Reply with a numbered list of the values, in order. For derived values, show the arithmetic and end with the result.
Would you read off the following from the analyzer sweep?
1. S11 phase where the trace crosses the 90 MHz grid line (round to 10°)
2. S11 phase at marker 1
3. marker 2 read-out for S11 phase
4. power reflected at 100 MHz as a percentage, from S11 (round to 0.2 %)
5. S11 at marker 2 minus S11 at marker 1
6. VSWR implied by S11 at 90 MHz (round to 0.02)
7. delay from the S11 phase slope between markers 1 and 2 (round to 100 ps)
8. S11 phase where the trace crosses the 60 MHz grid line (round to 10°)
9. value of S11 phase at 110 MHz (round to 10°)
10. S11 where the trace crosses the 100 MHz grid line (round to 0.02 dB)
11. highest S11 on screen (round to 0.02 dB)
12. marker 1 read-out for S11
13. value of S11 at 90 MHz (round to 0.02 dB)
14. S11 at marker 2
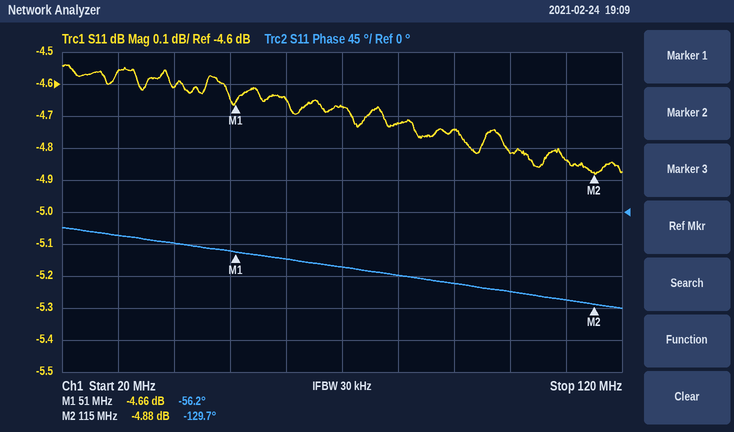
1. -100°
2. -56.2°
3. -129.7°
4. 10^(-4.82/10) ≈ 33.0 %
5. -4.88 − (-4.66) = -0.22 dB
6. |Γ| = 10^(-4.74/20) = 0.5794; VSWR = (1 + 0.5794)/(1 − 0.5794) ≈ 3.76
7. −(-129.7° − (-56.2°))/(360° × 64 MHz) ≈ 3.2 ns
8. -70°
9. -120°
10. -4.82 dB
11. -4.54 dB
12. -4.66 dB
13. -4.74 dB
14. -4.88 dB
